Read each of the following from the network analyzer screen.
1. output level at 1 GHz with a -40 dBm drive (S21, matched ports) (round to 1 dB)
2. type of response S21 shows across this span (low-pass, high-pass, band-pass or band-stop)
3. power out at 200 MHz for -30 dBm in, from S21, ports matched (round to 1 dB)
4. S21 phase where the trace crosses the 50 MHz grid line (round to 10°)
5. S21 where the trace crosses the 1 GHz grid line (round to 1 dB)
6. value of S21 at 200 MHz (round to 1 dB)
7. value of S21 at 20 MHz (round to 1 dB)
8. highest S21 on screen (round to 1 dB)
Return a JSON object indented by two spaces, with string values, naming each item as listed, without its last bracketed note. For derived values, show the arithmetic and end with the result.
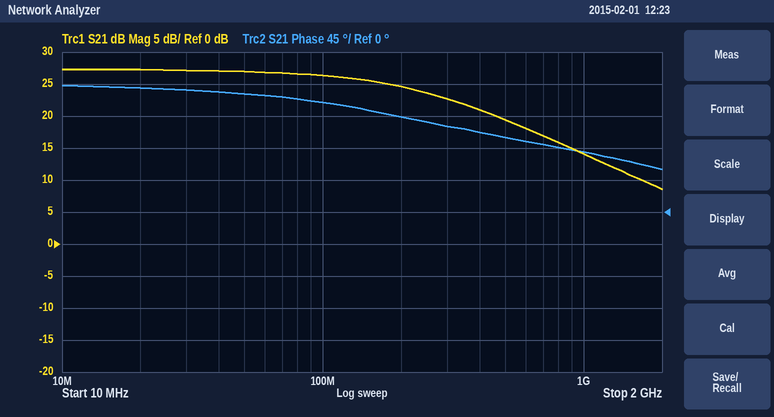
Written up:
{
  "output level at 1 GHz with a -40 dBm drive (S21, matched ports)": "-40 dBm + (14 dB) = -26 dBm",
  "type of response S21 shows across this span": "low-pass",
  "power out at 200 MHz for -30 dBm in, from S21, ports matched": "-30 dBm + (25 dB) = -5 dBm",
  "S21 phase where the trace crosses the 50 MHz grid line": "170°",
  "S21 where the trace crosses the 1 GHz grid line": "14 dB",
  "value of S21 at 200 MHz": "25 dB",
  "value of S21 at 20 MHz": "27 dB",
  "highest S21 on screen": "27 dB"
}
